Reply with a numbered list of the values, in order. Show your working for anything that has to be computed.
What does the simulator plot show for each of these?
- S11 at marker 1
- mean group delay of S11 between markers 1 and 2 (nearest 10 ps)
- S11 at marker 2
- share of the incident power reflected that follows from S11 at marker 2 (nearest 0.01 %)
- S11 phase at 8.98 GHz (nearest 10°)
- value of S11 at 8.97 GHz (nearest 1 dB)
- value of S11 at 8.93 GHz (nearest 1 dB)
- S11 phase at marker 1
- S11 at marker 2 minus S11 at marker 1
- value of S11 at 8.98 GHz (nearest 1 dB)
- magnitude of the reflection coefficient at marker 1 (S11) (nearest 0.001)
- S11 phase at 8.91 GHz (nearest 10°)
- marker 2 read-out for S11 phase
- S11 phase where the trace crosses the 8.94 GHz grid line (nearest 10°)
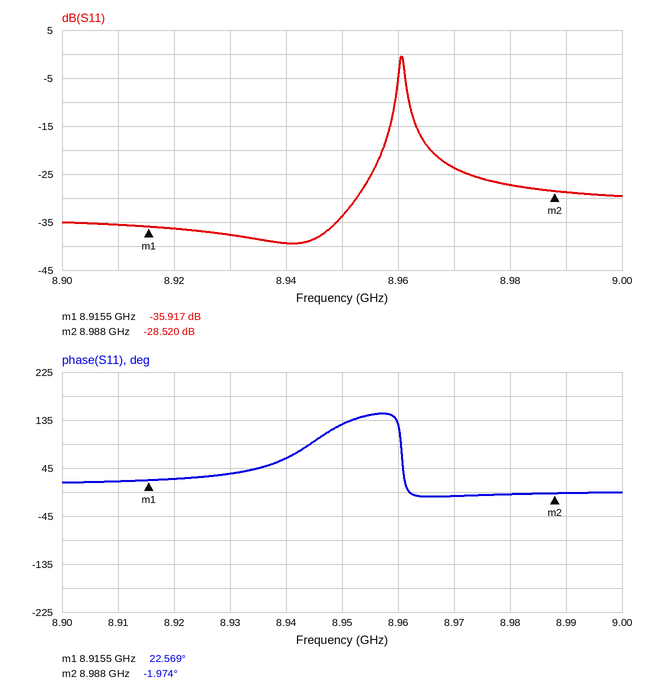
1. -35.917 dB
2. −(-1.974° − (22.569°))/(360° × 72.5 MHz) ≈ 940 ps
3. -28.520 dB
4. 10^(-28.52/10) ≈ 0.14 %
5. 0°
6. -24 dB
7. -38 dB
8. 22.569°
9. -28.52 − (-35.917) = 7.397 dB
10. -27 dB
11. 10^(-35.917/20) ≈ 0.016
12. 20°
13. -1.974°
14. 60°
